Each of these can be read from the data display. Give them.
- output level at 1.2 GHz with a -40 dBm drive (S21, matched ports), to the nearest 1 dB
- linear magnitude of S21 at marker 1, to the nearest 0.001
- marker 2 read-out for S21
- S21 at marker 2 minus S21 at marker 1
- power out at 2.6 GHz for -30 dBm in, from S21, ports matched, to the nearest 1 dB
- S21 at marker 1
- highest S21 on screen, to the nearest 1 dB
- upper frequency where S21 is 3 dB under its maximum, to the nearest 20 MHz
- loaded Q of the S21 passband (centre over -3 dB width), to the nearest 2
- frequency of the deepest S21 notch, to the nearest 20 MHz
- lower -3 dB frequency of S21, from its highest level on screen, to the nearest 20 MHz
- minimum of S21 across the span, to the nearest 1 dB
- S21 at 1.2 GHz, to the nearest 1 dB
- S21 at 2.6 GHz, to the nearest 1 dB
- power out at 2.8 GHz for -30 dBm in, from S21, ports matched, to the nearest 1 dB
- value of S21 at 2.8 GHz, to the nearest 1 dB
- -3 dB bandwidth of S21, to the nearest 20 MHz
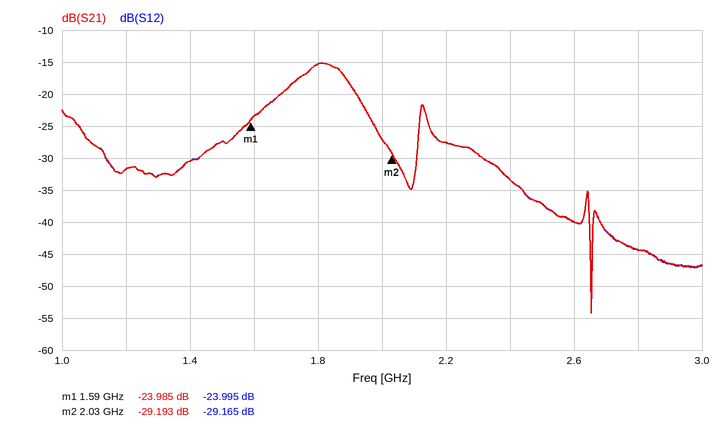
-72 dBm
0.063
-29.193 dB
-5.208 dB
-70 dBm
-23.985 dB
-15 dB
1.90 GHz
10
2.66 GHz
1.72 GHz
-54 dB
-32 dB
-40 dB
-74 dBm
-44 dB
180 MHz
